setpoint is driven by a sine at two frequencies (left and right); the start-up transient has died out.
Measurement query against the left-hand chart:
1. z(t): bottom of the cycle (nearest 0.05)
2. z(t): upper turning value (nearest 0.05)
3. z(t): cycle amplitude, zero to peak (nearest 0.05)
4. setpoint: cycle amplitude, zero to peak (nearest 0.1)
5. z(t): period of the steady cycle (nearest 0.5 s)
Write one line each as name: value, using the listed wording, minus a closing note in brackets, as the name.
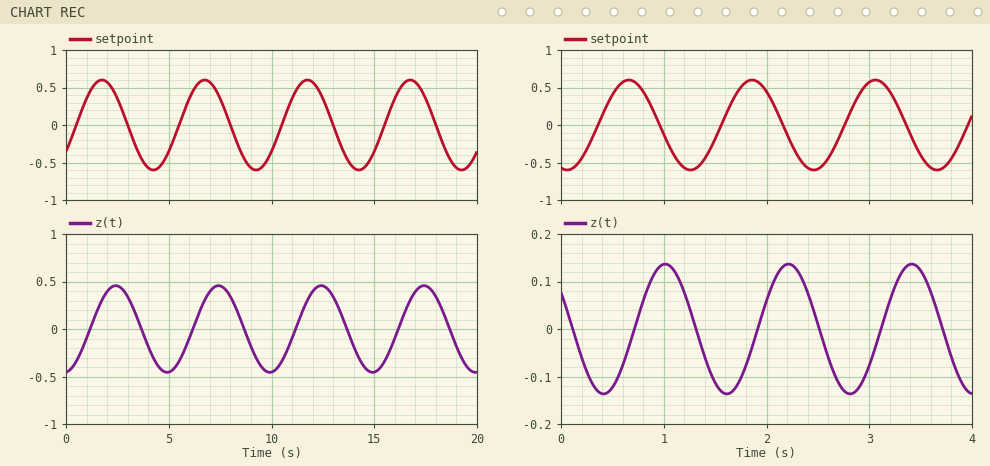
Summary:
z(t): bottom of the cycle: -0.45
z(t): upper turning value: 0.45
z(t): cycle amplitude, zero to peak: 0.45
setpoint: cycle amplitude, zero to peak: 0.6
z(t): period of the steady cycle: 5.0 s
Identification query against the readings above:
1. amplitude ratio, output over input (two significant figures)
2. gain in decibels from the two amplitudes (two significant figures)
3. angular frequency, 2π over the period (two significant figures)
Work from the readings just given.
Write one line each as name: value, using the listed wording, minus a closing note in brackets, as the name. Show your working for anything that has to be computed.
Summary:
amplitude ratio, output over input: 0.45 / 0.6 = 0.75
gain in decibels from the two amplitudes: 20 log10(0.45 / 0.6) = -2.5 dB
angular frequency, 2π over the period: 2π / 5 = 1.3 rad/s
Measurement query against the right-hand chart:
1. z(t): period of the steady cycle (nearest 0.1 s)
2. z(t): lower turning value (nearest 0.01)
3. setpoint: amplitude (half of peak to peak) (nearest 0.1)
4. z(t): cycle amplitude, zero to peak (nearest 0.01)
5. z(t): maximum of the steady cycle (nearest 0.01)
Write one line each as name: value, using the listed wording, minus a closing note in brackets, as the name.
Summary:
z(t): period of the steady cycle: 1.2 s
z(t): lower turning value: -0.14
setpoint: amplitude (half of peak to peak): 0.6
z(t): cycle amplitude, zero to peak: 0.14
z(t): maximum of the steady cycle: 0.14
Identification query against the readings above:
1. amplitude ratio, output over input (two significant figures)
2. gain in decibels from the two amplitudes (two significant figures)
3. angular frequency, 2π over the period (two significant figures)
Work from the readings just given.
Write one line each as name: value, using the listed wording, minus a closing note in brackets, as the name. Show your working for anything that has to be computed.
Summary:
amplitude ratio, output over input: 0.14 / 0.6 = 0.23
gain in decibels from the two amplitudes: 20 log10(0.14 / 0.6) = -13 dB
angular frequency, 2π over the period: 2π / 1.2 = 5.2 rad/s
